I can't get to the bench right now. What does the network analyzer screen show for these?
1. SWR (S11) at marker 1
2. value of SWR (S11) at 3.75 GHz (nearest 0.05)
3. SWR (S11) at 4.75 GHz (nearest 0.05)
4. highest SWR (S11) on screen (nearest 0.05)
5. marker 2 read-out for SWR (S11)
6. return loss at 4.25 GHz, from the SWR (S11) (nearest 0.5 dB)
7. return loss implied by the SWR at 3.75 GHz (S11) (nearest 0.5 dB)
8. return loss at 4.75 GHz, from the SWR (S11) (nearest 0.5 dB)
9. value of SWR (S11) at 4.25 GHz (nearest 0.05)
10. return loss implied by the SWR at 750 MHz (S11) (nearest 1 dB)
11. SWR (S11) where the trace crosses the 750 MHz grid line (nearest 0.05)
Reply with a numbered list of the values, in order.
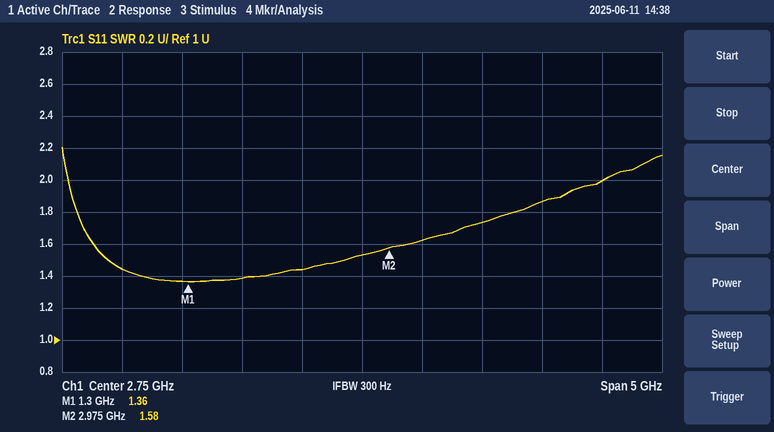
1. 1.36
2. 1.75
3. 2.00
4. 2.20
5. 1.58
6. 10.5 dB
7. 11.5 dB
8. 9.5 dB
9. 1.85
10. 15 dB
11. 1.45
